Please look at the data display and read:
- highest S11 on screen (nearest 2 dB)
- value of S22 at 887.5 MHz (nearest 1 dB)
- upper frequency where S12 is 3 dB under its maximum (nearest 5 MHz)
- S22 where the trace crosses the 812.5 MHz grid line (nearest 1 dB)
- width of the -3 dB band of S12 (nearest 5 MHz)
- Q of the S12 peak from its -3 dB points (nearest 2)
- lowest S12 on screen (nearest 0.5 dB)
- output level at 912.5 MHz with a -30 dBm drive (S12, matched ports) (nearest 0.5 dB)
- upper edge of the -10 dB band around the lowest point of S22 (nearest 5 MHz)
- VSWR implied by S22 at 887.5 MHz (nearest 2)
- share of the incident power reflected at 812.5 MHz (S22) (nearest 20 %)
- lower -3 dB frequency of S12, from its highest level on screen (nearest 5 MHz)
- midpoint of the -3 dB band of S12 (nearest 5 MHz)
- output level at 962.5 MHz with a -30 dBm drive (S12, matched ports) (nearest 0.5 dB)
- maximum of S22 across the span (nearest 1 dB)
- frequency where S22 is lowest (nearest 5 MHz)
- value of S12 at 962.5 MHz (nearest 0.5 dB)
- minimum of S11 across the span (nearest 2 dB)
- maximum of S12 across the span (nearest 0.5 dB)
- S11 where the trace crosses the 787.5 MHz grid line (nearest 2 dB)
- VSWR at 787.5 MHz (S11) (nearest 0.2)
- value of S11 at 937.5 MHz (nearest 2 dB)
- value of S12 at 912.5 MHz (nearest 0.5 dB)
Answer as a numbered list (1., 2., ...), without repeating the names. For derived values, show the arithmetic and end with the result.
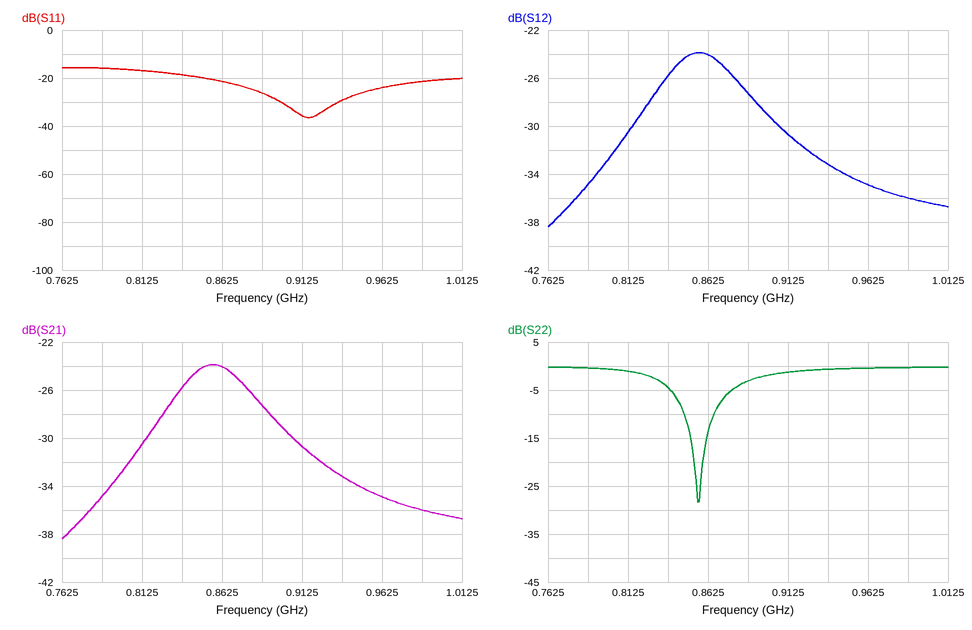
1. -16 dB
2. -3 dB
3. 885 MHz
4. -1 dB
5. 885 MHz − 830 MHz = 55 MHz
6. 857.5 MHz / 55 MHz ≈ 16
7. -38.5 dB
8. -30 dBm + (-30.5 dB) = -60.5 dBm
9. 865 MHz
10. |Γ| = 10^(-3/20) = 0.7079; VSWR = (1 + 0.7079)/(1 − 0.7079) ≈ 6
11. 10^(-1/10) ≈ 79.4 %, so 80 % to the nearest 20 %
12. 830 MHz
13. 860 MHz
14. -30 dBm + (-35.0 dB) = -65.0 dBm
15. 0 dB
16. 855 MHz
17. -35.0 dB
18. -36 dB
19. -24.0 dB
20. -16 dB
21. |Γ| = 10^(-16/20) = 0.1585; VSWR = (1 + 0.1585)/(1 − 0.1585) ≈ 1.4
22. -30 dB
23. -30.5 dB
